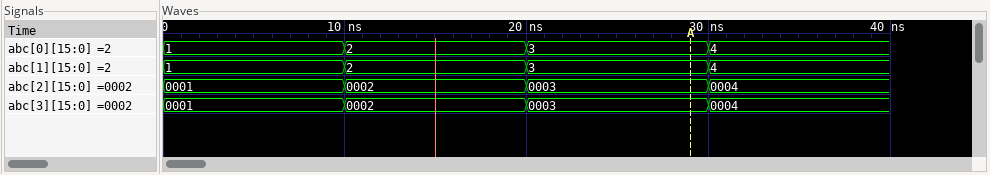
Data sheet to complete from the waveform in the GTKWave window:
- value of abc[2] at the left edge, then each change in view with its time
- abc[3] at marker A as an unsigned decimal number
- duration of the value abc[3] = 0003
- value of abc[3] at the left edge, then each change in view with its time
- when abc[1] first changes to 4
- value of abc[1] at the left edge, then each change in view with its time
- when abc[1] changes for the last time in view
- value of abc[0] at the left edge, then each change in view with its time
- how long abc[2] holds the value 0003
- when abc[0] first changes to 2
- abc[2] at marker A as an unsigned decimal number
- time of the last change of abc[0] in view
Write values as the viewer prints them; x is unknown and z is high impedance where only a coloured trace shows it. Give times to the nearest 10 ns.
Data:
0001, 0002 at 10 ns, 0003 at 20 ns, 0004 at 30 ns
3
10 ns
0001, 0002 at 10 ns, 0003 at 20 ns, 0004 at 30 ns
30 ns
1, 2 at 10 ns, 3 at 20 ns, 4 at 30 ns
30 ns
1, 2 at 10 ns, 3 at 20 ns, 4 at 30 ns
10 ns
10 ns
3
30 ns
